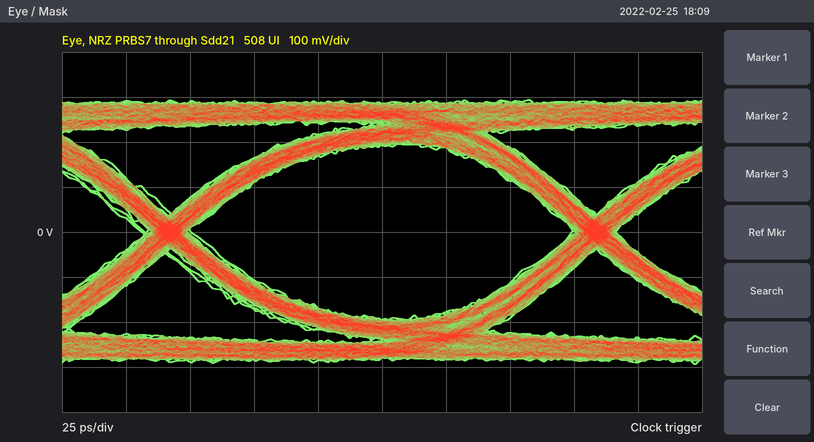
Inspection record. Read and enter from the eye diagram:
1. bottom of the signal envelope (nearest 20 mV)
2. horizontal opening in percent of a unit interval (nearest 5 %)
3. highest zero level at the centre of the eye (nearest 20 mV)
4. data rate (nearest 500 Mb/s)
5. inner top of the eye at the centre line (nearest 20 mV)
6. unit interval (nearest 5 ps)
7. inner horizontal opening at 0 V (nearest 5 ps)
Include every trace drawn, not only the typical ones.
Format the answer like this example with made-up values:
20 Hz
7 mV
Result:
-300 mV
90 %
-200 mV
6.0 Gb/s
200 mV
165 ps
150 ps
